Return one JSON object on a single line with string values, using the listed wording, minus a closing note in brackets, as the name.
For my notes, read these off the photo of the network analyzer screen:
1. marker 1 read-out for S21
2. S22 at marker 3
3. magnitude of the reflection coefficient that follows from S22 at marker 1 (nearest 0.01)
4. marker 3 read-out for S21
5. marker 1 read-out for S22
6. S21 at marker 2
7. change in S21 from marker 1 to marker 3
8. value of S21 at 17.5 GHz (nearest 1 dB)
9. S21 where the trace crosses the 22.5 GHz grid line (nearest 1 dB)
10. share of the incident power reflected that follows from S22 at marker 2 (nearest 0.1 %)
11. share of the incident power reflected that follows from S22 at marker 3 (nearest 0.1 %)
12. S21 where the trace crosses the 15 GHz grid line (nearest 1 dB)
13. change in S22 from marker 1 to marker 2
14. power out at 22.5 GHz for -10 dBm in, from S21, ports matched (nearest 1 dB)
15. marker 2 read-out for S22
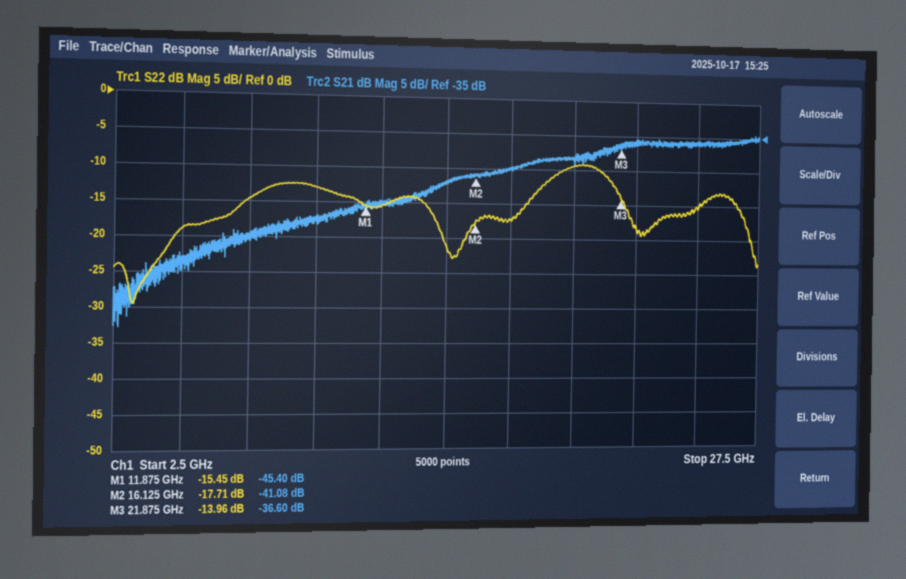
{"marker 1 read-out for S21": "-45.40 dB", "S22 at marker 3": "-13.96 dB", "magnitude of the reflection coefficient that follows from S22 at marker 1": "0.17", "marker 3 read-out for S21": "-36.60 dB", "marker 1 read-out for S22": "-15.45 dB", "S21 at marker 2": "-41.08 dB", "change in S21 from marker 1 to marker 3": "8.80 dB", "value of S21 at 17.5 GHz": "-40 dB", "S21 where the trace crosses the 22.5 GHz grid line": "-36 dB", "share of the incident power reflected that follows from S22 at marker 2": "1.7 %", "share of the incident power reflected that follows from S22 at marker 3": "4.0 %", "S21 where the trace crosses the 15 GHz grid line": "-42 dB", "change in S22 from marker 1 to marker 2": "-2.26 dB", "power out at 22.5 GHz for -10 dBm in, from S21, ports matched": "-46 dBm", "marker 2 read-out for S22": "-17.71 dB"}
